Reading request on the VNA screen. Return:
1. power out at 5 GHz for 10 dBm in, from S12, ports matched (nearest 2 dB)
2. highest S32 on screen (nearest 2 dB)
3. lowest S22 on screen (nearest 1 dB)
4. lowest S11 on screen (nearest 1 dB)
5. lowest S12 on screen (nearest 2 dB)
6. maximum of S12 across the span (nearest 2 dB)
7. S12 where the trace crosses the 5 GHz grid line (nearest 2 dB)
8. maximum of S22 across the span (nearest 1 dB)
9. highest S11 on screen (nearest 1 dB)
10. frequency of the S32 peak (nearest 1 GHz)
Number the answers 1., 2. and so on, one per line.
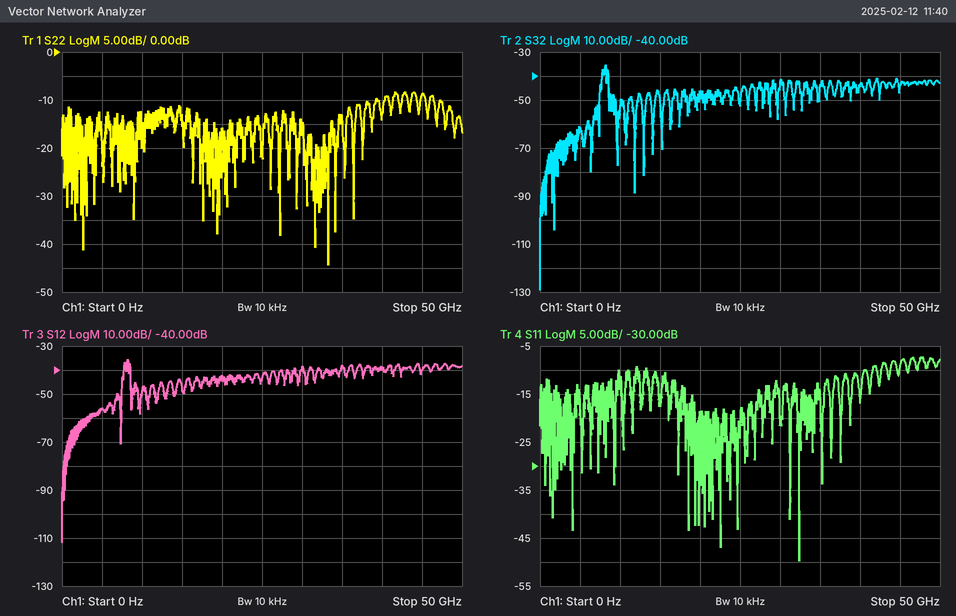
1. -46 dBm
2. -36 dB
3. -44 dB
4. -50 dB
5. -112 dB
6. -36 dB
7. -56 dB
8. -8 dB
9. -7 dB
10. 8 GHz
